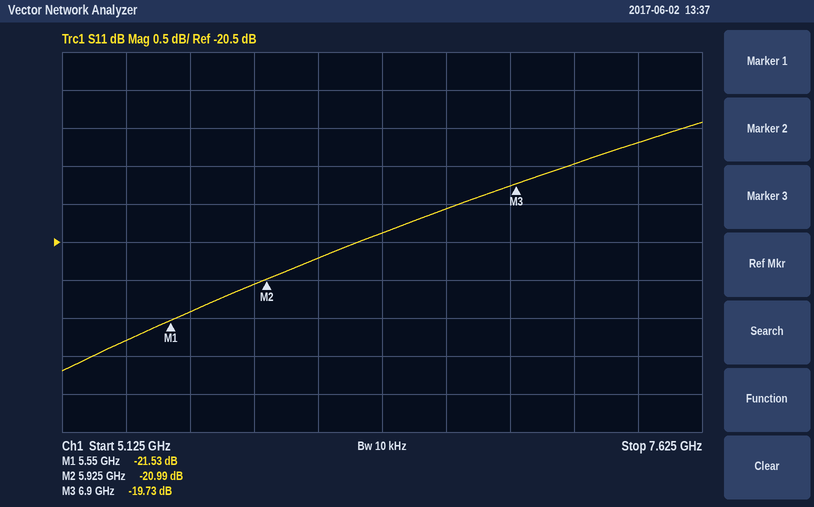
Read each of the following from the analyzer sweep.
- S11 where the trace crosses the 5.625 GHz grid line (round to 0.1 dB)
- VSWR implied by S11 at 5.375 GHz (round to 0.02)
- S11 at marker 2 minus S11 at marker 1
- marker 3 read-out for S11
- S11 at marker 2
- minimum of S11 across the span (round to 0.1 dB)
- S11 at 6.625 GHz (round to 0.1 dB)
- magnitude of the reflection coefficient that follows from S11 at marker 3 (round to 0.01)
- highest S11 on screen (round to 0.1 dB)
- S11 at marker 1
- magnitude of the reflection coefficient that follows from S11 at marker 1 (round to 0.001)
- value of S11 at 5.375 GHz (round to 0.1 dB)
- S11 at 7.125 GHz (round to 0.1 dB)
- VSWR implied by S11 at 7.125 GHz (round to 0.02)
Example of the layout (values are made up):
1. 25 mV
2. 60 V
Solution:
1. -21.4 dB
2. 1.18
3. 0.54 dB
4. -19.73 dB
5. -20.99 dB
6. -22.2 dB
7. -20.1 dB
8. 0.10
9. -18.9 dB
10. -21.53 dB
11. 0.084
12. -21.8 dB
13. -19.5 dB
14. 1.24
